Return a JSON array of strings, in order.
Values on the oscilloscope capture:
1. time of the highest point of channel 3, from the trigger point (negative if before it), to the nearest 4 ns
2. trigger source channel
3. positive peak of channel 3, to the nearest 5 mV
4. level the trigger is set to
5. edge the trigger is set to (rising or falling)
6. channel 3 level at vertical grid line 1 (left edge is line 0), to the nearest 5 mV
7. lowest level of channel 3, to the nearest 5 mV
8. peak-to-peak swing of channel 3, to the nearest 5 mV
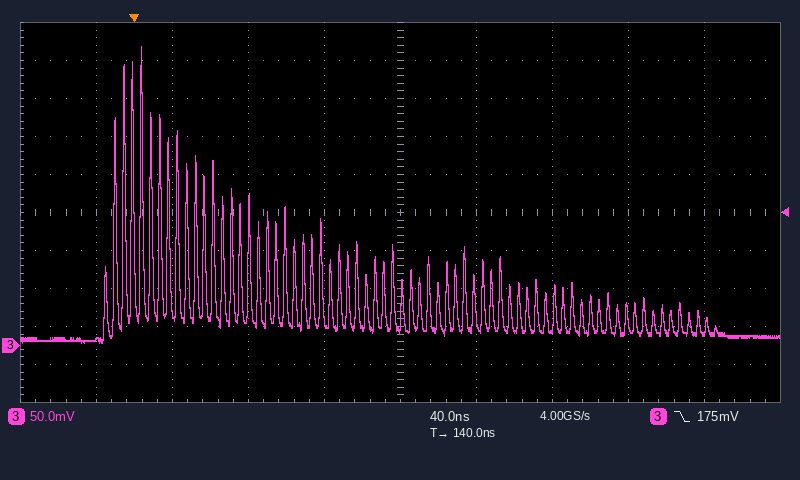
["+4 ns", "channel 3", "395 mV", "175 mV", "falling", "5 mV", "5 mV", "390 mV"]
